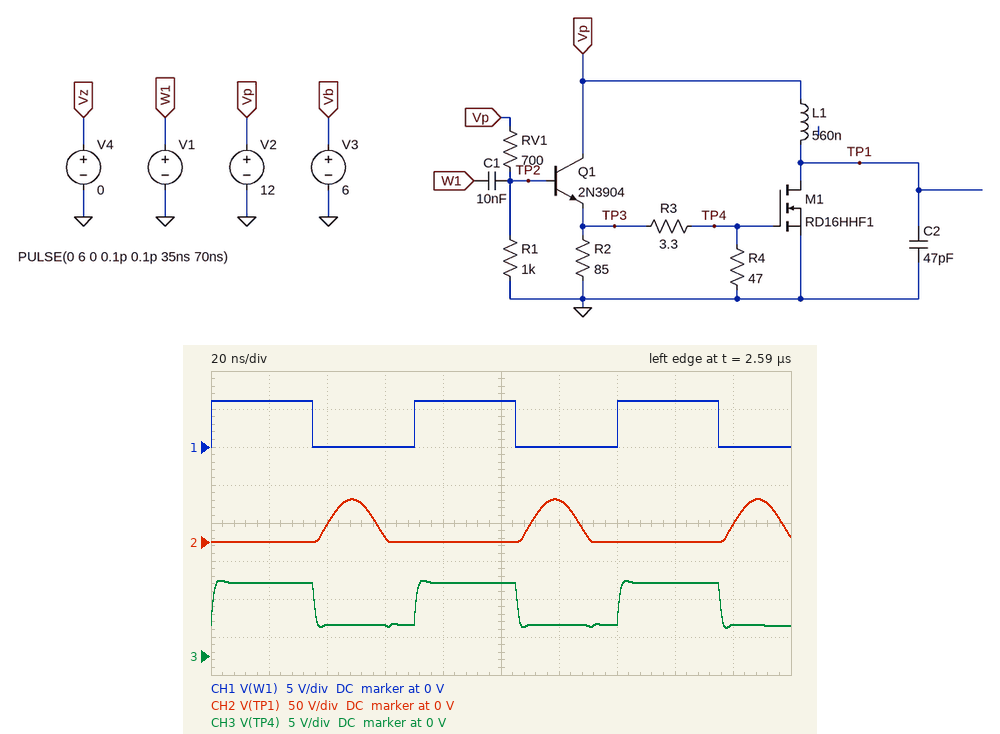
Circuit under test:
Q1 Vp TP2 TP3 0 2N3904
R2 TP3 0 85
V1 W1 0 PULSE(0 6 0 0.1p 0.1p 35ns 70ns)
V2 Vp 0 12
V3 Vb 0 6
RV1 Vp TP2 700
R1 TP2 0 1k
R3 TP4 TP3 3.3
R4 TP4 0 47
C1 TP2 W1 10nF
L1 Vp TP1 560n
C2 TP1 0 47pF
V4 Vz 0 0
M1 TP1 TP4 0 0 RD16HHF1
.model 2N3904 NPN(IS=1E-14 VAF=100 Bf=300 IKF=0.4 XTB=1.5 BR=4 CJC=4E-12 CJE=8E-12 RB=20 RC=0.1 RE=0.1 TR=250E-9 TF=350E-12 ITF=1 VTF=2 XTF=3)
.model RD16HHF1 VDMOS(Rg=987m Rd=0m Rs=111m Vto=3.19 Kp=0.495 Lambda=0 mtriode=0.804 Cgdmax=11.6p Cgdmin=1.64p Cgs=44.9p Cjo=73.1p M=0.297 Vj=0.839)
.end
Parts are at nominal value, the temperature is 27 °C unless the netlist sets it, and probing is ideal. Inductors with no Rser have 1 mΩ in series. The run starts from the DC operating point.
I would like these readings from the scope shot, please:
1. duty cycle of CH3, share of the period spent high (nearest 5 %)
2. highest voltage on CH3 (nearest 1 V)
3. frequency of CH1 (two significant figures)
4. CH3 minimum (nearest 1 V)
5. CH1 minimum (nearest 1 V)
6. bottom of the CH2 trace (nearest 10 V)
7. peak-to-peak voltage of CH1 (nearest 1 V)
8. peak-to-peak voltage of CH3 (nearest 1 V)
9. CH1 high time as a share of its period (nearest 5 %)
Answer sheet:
50 %
10 V
14 MHz
4 V
0 V
0 V
6 V
6 V
50 %
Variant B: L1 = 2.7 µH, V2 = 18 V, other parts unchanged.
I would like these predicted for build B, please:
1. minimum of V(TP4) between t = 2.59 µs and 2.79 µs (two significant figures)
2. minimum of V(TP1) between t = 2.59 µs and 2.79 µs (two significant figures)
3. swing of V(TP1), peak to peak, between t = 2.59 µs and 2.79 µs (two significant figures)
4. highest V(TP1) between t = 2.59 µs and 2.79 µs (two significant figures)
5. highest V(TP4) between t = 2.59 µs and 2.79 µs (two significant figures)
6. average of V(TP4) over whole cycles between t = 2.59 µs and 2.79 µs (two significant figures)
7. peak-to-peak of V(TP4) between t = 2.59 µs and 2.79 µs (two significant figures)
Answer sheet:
6.8 V
1.1 V
50 V
51 V
13 V
9.8 V
6.5 V
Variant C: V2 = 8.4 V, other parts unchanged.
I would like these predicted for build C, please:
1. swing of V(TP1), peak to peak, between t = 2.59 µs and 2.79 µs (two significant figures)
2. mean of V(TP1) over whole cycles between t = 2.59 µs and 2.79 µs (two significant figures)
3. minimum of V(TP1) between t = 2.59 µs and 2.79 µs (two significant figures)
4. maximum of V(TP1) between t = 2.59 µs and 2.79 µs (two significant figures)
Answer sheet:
40 V
8.4 V
-810 mV
39 V
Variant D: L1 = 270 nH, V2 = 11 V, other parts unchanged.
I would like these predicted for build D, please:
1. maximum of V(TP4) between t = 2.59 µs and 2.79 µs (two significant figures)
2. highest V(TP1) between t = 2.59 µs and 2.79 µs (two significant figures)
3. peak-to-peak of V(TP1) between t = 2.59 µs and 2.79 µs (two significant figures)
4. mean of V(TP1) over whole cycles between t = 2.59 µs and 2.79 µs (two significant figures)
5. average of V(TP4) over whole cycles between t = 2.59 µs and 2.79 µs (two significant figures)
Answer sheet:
9.4 V
81 V
82 V
11 V
6.3 V
